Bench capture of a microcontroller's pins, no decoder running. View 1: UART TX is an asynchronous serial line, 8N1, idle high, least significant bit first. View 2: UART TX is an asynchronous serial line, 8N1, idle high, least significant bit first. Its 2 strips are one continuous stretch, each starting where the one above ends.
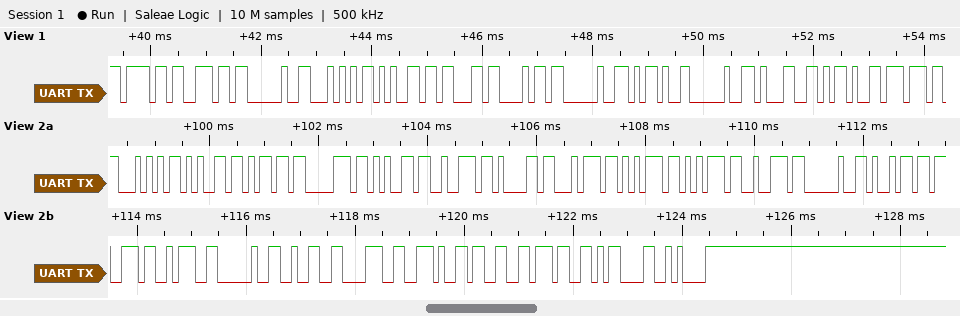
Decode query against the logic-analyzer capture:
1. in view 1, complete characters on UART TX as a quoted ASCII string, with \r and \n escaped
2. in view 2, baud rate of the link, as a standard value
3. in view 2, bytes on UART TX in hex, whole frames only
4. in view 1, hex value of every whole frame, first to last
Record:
"on Tech - 1-w"
9600 baud
54 65 6D 70 65 72 61 74 75 75 72 20 69 73 3A 20 32 38 2E 33 37 0D 0A
6F 6E 20 54 65 63 68 20 2D 20 31 2D 77
